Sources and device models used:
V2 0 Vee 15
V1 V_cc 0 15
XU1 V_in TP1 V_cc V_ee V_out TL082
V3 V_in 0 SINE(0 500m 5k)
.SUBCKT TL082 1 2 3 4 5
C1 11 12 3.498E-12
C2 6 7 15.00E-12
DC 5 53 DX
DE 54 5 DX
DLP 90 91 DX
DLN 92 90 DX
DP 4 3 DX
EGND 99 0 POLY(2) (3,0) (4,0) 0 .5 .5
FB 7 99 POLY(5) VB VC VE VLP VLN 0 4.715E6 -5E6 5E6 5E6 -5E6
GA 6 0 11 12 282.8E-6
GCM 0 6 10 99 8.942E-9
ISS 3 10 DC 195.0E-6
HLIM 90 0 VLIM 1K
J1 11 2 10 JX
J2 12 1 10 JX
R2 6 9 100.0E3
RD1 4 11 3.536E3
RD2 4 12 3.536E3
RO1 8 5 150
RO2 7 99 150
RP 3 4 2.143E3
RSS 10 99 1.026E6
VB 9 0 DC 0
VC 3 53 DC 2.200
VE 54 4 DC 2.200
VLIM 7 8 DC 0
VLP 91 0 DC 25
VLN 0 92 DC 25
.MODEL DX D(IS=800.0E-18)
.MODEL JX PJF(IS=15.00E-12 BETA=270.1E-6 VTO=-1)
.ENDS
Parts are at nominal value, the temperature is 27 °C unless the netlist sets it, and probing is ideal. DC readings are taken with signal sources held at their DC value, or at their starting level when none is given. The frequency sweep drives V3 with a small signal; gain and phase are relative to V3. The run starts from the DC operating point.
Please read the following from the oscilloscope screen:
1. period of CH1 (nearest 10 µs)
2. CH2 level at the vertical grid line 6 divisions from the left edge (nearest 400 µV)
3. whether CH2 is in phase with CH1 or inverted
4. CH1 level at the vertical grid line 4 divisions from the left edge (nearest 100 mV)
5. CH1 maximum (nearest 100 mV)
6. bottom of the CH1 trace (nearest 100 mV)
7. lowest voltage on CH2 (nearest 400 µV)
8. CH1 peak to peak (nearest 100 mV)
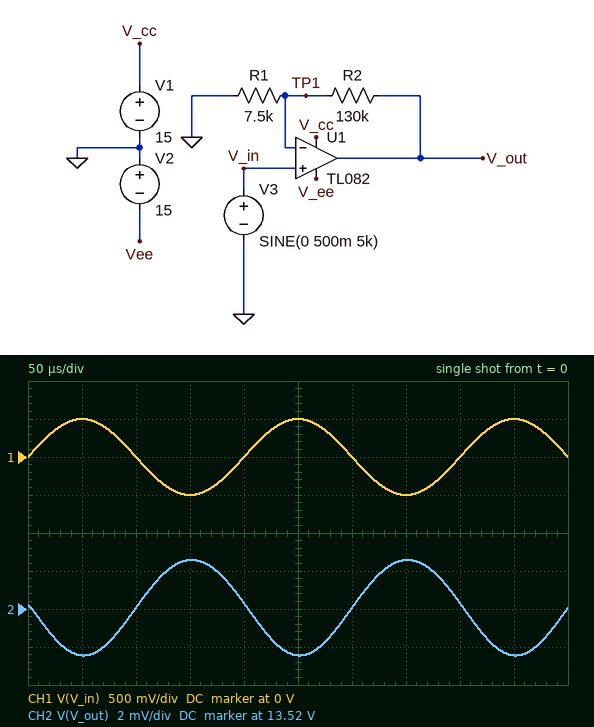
200 µs
13.5220 V
inverted
0 V
500 mV
-500 mV
13.5196 V
1.0 V
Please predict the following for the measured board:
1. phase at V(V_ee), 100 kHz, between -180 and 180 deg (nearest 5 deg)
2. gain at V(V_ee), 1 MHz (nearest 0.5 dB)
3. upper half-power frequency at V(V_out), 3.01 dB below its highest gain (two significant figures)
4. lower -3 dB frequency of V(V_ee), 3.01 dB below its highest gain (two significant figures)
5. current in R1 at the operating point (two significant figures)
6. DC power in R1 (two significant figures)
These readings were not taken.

0 deg
-9.5 dB
110 kHz
8.0 MHz
540 µA
2.2 mW
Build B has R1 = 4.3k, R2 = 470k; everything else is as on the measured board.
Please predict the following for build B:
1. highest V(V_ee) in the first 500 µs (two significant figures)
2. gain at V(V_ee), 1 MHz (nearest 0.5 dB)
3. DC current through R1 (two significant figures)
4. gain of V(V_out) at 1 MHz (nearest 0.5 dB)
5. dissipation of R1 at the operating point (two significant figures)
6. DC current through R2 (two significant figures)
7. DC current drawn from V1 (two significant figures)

8.0 V
-10.0 dB
700 µA
-62.5 dB
2.1 mW
22 µA
2.7 mA
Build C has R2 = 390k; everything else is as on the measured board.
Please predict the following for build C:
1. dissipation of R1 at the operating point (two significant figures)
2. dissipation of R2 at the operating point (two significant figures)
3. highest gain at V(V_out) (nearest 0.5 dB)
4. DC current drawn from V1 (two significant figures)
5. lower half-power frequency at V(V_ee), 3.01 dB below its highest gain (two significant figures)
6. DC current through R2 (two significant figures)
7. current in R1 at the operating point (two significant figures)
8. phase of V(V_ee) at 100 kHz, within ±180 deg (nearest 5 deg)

2.0 mW
240 µW
-45.5 dB
2.4 mA
7.8 MHz
25 µA
520 µA
0 deg
